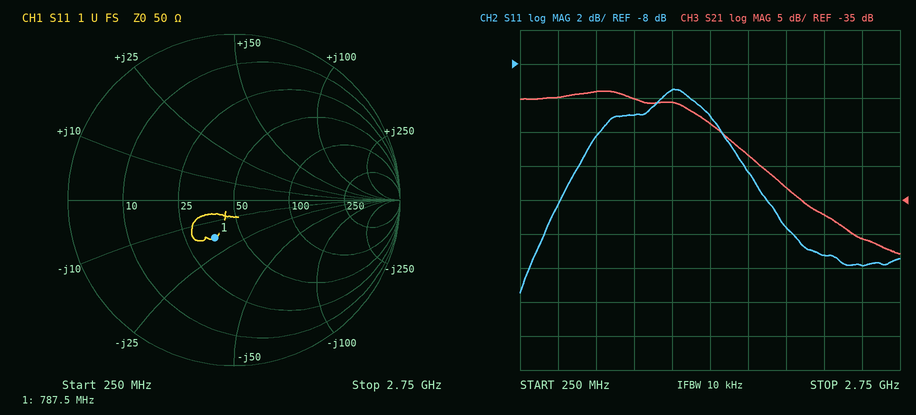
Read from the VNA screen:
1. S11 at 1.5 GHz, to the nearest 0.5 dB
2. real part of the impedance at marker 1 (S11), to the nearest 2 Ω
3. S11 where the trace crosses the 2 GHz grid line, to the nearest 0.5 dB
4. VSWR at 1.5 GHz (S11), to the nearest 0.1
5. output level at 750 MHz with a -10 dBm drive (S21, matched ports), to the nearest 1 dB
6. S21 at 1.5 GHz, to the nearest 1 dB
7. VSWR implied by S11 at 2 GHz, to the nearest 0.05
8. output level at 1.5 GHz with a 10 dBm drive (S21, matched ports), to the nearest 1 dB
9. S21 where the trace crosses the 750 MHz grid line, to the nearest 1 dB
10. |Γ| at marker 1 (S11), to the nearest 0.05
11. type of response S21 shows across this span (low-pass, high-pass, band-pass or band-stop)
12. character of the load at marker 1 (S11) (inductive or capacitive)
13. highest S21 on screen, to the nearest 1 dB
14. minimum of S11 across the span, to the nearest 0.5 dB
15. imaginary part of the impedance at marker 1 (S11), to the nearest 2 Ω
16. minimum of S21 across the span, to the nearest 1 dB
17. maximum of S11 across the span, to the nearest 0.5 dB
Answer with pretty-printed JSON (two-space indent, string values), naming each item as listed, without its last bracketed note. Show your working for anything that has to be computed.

{
  "S11 at 1.5 GHz, to the nearest 0.5 dB": "-11.0 dB",
  "real part of the impedance at marker 1 (S11), to the nearest 2 Ω": "36 Ω",
  "S11 where the trace crosses the 2 GHz grid line, to the nearest 0.5 dB": "-17.5 dB",
  "VSWR at 1.5 GHz (S11), to the nearest 0.1": "|Γ| = 10^(-11/20) = 0.2818; VSWR = (1 + 0.2818)/(1 − 0.2818) ≈ 1.8",
  "output level at 750 MHz with a -10 dBm drive (S21, matched ports), to the nearest 1 dB": "-10 dBm + (-19 dB) = -29 dBm",
  "S21 at 1.5 GHz, to the nearest 1 dB": "-24 dB",
  "VSWR implied by S11 at 2 GHz, to the nearest 0.05": "|Γ| = 10^(-17.5/20) = 0.1334; VSWR = (1 + 0.1334)/(1 − 0.1334) ≈ 1.31, so 1.30 to the nearest 0.05",
  "output level at 1.5 GHz with a 10 dBm drive (S21, matched ports), to the nearest 1 dB": "10 dBm + (-24 dB) = -14 dBm",
  "S21 where the trace crosses the 750 MHz grid line, to the nearest 1 dB": "-19 dB",
  "|Γ| at marker 1 (S11), to the nearest 0.05": "0.25",
  "type of response S21 shows across this span": "low-pass",
  "character of the load at marker 1 (S11)": "capacitive",
  "highest S21 on screen, to the nearest 1 dB": "-19 dB",
  "minimum of S11 across the span, to the nearest 0.5 dB": "-21.5 dB",
  "imaginary part of the impedance at marker 1 (S11), to the nearest 2 Ω": "-18 Ω",
  "minimum of S21 across the span, to the nearest 1 dB": "-43 dB",
  "maximum of S11 across the span, to the nearest 0.5 dB": "-9.5 dB"
}
